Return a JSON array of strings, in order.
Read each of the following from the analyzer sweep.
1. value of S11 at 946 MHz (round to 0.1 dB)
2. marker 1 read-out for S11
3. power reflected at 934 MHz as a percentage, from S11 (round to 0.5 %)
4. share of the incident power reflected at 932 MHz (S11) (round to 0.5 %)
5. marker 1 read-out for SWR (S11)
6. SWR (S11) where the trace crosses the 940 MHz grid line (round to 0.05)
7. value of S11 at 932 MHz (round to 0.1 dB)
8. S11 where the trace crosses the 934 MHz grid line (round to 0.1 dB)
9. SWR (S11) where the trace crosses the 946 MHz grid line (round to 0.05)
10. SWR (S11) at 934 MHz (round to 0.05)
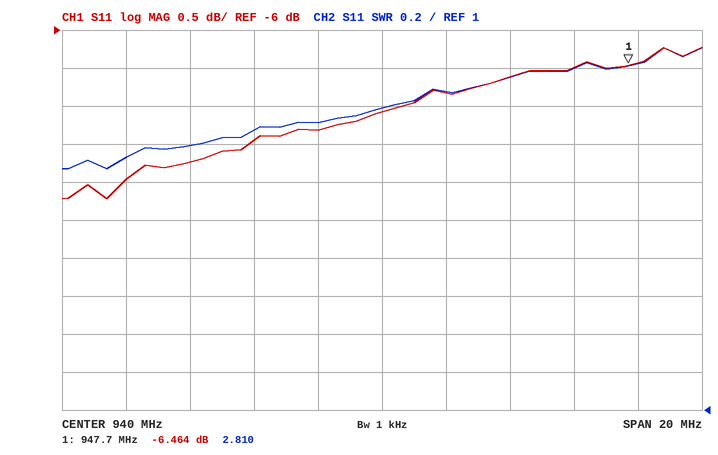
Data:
["-6.5 dB", "-6.464 dB", "17.0 %", "16.0 %", "2.810", "2.60", "-8.0 dB", "-7.7 dB", "2.80", "2.40"]
